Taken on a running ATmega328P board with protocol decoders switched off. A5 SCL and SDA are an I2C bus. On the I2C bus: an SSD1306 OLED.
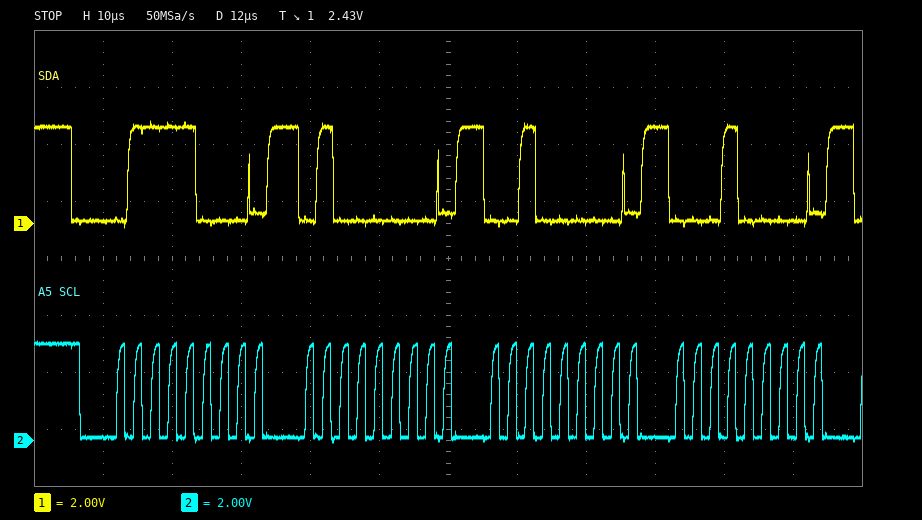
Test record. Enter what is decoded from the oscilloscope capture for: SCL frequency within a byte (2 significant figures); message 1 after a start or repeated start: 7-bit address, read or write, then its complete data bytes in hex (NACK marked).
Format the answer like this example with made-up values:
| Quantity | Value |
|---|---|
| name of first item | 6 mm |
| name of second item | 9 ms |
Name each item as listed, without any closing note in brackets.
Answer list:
| Quantity | Value |
|---|---|
| SCL frequency within a byte | 400 kHz |
| message 1 after a start or repeated start: 7-bit address, read or write, then its complete data bytes in hex | 0x3C write: 40 20 10 |
